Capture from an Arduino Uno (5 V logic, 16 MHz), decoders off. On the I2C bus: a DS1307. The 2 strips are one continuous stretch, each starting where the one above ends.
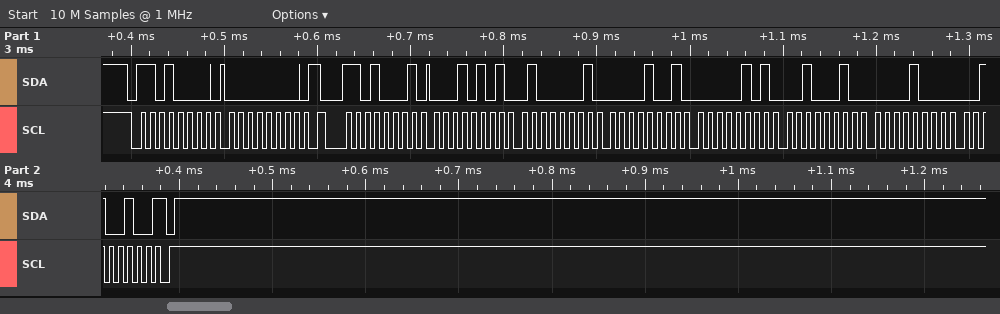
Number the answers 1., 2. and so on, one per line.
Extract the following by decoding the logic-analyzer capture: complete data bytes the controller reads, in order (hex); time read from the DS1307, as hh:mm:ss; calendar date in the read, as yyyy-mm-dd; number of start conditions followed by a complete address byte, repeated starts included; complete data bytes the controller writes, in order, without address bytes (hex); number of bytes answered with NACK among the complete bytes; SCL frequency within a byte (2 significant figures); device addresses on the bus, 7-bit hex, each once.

1. 15 41 09 05 22 08 24
2. 09:41:15
3. 2024-08-22
4. 2
5. 00
6. 1
7. 100 kHz
8. 0x68
